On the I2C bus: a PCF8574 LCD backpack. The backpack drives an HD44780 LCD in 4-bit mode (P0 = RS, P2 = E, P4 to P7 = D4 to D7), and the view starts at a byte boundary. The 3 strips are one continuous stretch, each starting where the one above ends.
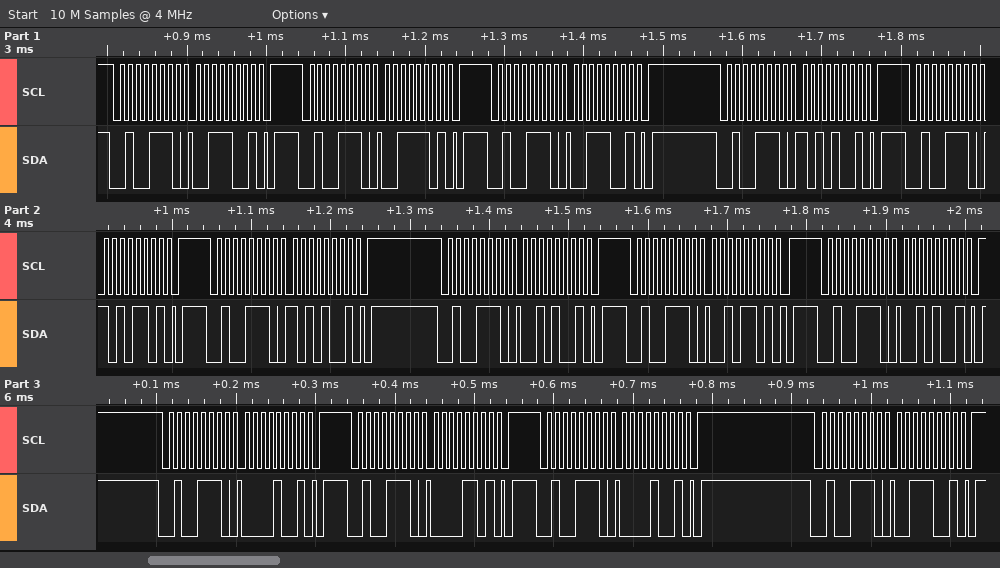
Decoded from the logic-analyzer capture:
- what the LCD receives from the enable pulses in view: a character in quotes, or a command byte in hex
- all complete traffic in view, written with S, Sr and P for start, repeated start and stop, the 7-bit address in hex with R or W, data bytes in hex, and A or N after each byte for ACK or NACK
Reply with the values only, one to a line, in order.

':' ' '
S 27W A 39 A P S 27W A 3D A P S 27W A 39 A P S 27W A A9 A P S 27W A AD A P S 27W A A9 A P S 27W A 29 A P S 27W A 2D A P S 27W A 29 A P S 27W A 09 A P S 27W A 0D A P S 27W A 09 A P S 27W A 39 A P
